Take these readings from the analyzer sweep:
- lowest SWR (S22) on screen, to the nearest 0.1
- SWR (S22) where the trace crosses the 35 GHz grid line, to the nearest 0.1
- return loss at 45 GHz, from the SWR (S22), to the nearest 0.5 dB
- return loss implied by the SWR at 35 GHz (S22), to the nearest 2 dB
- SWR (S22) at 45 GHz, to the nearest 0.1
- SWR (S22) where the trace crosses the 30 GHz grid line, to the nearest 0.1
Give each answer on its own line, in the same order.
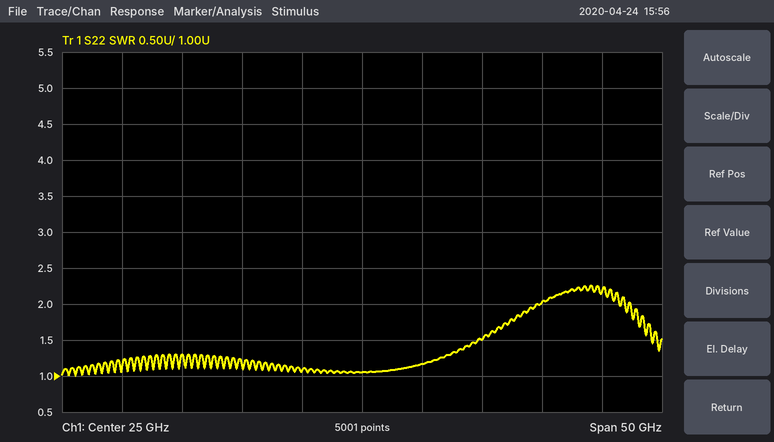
1.0
1.5
8.5 dB
14 dB
2.2
1.2
